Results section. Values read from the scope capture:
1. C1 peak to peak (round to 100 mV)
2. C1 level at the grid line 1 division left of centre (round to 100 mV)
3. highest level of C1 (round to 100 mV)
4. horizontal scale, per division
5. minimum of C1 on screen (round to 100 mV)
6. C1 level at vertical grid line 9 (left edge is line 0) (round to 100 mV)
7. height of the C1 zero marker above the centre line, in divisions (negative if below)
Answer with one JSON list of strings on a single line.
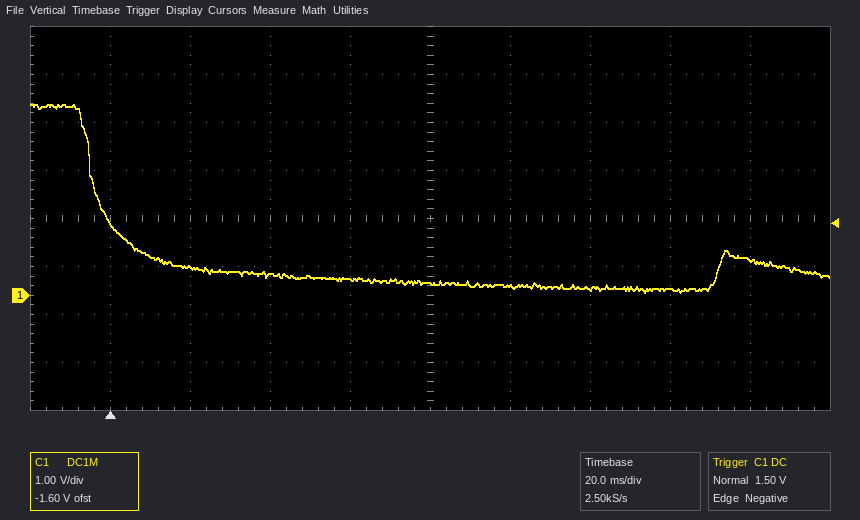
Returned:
["3.9 V", "300 mV", "4.0 V", "20 ms", "100 mV", "700 mV", "-1.6 div"]
